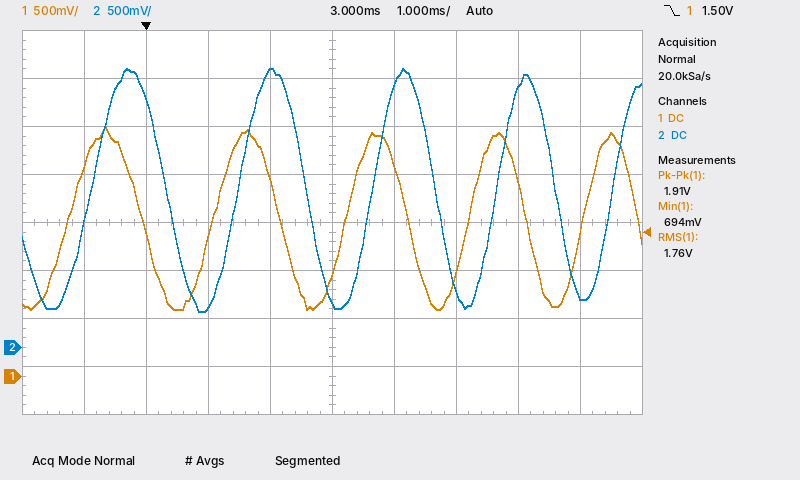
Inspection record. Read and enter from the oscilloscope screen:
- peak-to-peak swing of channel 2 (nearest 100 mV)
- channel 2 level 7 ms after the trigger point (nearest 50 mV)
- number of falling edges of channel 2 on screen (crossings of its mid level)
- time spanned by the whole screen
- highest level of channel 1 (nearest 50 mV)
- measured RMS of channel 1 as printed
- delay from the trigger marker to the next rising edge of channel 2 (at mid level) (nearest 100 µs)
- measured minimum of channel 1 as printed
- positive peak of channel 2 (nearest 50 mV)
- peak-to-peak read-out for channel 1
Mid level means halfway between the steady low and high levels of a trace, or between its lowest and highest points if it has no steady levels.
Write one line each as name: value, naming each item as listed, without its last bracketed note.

peak-to-peak swing of channel 2: 2.50 V
channel 2 level 7 ms after the trigger point: 550 mV
number of falling edges of channel 2 on screen: 4
time spanned by the whole screen: 10 ms
highest level of channel 1: 2.60 V
measured RMS of channel 1 as printed: 1.76 V
delay from the trigger marker to the next rising edge of channel 2 (at mid level): 1.5 ms
measured minimum of channel 1 as printed: 694 mV
positive peak of channel 2: 2.90 V
peak-to-peak read-out for channel 1: 1.91 V
